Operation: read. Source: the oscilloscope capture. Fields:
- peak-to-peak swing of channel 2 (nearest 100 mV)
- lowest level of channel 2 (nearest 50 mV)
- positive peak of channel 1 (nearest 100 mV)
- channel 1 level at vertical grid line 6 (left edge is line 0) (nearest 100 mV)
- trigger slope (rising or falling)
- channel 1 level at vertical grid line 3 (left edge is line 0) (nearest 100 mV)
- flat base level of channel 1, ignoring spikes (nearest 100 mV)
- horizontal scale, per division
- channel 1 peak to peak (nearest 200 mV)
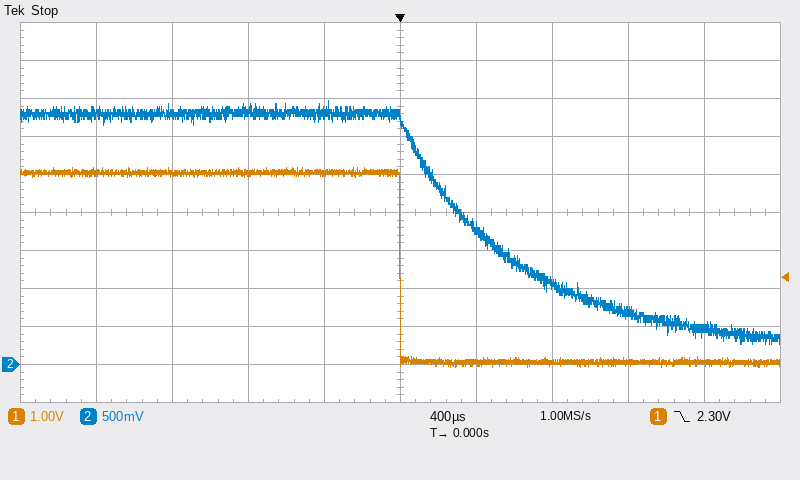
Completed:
3.20 V
300 mV
5.2 V
100 mV
falling
5.0 V
100 mV
400 µs
5.2 V
